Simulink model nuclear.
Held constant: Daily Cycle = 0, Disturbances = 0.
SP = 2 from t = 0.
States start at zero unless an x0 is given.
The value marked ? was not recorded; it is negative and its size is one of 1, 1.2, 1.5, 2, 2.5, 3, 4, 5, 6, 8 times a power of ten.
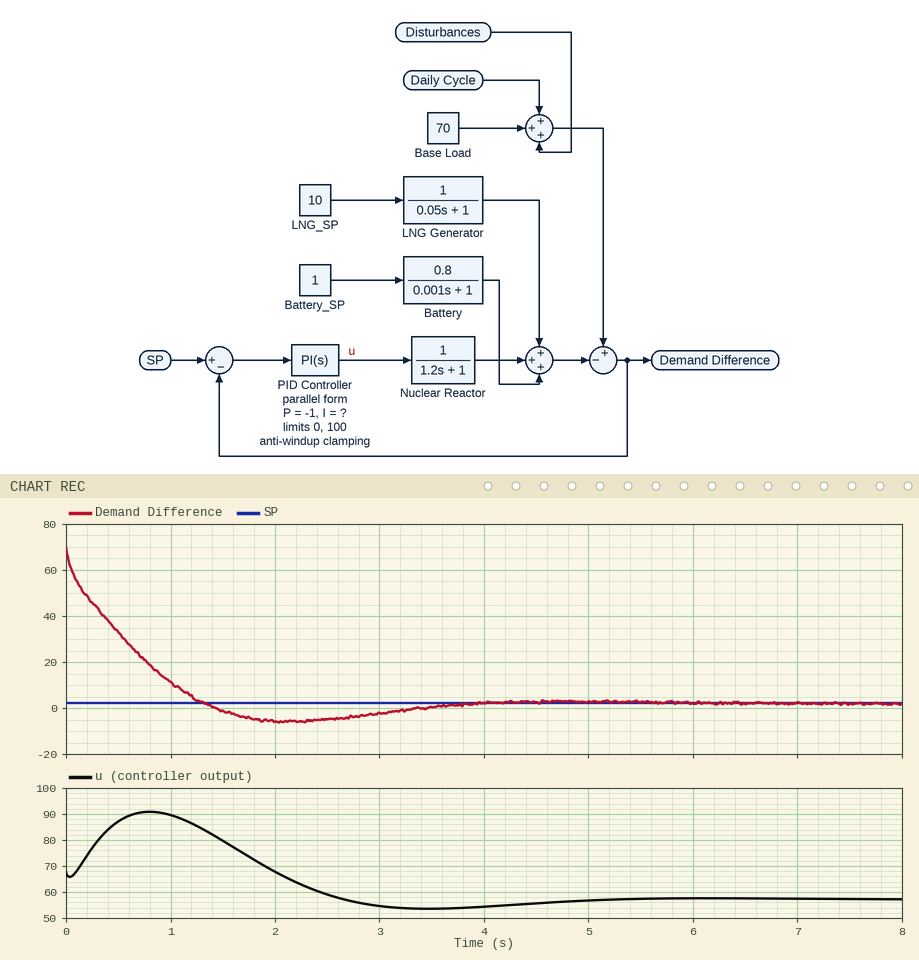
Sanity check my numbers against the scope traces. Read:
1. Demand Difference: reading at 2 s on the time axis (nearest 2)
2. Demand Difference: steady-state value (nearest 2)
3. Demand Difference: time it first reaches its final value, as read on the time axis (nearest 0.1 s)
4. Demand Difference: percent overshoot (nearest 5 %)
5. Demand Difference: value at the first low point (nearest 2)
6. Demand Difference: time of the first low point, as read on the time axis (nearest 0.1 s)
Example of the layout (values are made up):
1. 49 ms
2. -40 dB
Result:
1. -6
2. 2
3. 1.3 s
4. 10 %
5. -6
6. 2.1 s
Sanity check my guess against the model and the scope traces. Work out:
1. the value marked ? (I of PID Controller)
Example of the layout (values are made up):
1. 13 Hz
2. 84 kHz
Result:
1. -2.5
